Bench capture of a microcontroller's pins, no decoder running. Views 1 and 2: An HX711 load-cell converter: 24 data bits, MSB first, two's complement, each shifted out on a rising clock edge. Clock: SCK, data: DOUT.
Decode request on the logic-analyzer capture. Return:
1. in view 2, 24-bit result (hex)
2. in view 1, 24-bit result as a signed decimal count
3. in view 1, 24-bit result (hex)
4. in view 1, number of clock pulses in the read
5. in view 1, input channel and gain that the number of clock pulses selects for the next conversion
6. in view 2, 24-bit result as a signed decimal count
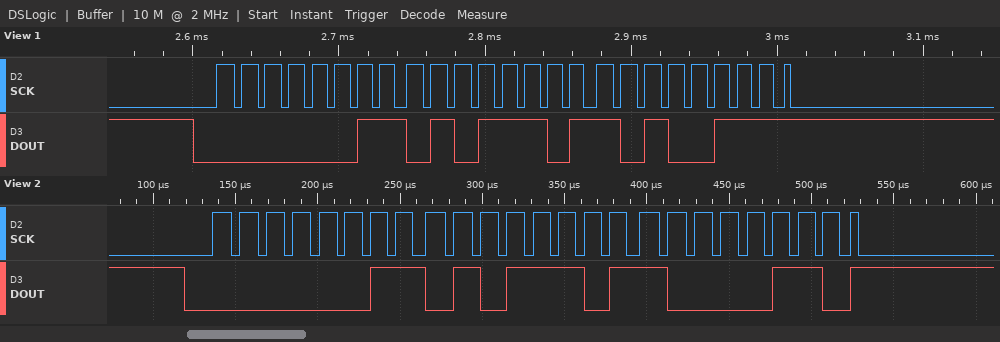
0x035D86
220583
0x035DA7
25
channel A, gain 128
220550
